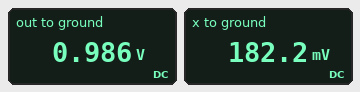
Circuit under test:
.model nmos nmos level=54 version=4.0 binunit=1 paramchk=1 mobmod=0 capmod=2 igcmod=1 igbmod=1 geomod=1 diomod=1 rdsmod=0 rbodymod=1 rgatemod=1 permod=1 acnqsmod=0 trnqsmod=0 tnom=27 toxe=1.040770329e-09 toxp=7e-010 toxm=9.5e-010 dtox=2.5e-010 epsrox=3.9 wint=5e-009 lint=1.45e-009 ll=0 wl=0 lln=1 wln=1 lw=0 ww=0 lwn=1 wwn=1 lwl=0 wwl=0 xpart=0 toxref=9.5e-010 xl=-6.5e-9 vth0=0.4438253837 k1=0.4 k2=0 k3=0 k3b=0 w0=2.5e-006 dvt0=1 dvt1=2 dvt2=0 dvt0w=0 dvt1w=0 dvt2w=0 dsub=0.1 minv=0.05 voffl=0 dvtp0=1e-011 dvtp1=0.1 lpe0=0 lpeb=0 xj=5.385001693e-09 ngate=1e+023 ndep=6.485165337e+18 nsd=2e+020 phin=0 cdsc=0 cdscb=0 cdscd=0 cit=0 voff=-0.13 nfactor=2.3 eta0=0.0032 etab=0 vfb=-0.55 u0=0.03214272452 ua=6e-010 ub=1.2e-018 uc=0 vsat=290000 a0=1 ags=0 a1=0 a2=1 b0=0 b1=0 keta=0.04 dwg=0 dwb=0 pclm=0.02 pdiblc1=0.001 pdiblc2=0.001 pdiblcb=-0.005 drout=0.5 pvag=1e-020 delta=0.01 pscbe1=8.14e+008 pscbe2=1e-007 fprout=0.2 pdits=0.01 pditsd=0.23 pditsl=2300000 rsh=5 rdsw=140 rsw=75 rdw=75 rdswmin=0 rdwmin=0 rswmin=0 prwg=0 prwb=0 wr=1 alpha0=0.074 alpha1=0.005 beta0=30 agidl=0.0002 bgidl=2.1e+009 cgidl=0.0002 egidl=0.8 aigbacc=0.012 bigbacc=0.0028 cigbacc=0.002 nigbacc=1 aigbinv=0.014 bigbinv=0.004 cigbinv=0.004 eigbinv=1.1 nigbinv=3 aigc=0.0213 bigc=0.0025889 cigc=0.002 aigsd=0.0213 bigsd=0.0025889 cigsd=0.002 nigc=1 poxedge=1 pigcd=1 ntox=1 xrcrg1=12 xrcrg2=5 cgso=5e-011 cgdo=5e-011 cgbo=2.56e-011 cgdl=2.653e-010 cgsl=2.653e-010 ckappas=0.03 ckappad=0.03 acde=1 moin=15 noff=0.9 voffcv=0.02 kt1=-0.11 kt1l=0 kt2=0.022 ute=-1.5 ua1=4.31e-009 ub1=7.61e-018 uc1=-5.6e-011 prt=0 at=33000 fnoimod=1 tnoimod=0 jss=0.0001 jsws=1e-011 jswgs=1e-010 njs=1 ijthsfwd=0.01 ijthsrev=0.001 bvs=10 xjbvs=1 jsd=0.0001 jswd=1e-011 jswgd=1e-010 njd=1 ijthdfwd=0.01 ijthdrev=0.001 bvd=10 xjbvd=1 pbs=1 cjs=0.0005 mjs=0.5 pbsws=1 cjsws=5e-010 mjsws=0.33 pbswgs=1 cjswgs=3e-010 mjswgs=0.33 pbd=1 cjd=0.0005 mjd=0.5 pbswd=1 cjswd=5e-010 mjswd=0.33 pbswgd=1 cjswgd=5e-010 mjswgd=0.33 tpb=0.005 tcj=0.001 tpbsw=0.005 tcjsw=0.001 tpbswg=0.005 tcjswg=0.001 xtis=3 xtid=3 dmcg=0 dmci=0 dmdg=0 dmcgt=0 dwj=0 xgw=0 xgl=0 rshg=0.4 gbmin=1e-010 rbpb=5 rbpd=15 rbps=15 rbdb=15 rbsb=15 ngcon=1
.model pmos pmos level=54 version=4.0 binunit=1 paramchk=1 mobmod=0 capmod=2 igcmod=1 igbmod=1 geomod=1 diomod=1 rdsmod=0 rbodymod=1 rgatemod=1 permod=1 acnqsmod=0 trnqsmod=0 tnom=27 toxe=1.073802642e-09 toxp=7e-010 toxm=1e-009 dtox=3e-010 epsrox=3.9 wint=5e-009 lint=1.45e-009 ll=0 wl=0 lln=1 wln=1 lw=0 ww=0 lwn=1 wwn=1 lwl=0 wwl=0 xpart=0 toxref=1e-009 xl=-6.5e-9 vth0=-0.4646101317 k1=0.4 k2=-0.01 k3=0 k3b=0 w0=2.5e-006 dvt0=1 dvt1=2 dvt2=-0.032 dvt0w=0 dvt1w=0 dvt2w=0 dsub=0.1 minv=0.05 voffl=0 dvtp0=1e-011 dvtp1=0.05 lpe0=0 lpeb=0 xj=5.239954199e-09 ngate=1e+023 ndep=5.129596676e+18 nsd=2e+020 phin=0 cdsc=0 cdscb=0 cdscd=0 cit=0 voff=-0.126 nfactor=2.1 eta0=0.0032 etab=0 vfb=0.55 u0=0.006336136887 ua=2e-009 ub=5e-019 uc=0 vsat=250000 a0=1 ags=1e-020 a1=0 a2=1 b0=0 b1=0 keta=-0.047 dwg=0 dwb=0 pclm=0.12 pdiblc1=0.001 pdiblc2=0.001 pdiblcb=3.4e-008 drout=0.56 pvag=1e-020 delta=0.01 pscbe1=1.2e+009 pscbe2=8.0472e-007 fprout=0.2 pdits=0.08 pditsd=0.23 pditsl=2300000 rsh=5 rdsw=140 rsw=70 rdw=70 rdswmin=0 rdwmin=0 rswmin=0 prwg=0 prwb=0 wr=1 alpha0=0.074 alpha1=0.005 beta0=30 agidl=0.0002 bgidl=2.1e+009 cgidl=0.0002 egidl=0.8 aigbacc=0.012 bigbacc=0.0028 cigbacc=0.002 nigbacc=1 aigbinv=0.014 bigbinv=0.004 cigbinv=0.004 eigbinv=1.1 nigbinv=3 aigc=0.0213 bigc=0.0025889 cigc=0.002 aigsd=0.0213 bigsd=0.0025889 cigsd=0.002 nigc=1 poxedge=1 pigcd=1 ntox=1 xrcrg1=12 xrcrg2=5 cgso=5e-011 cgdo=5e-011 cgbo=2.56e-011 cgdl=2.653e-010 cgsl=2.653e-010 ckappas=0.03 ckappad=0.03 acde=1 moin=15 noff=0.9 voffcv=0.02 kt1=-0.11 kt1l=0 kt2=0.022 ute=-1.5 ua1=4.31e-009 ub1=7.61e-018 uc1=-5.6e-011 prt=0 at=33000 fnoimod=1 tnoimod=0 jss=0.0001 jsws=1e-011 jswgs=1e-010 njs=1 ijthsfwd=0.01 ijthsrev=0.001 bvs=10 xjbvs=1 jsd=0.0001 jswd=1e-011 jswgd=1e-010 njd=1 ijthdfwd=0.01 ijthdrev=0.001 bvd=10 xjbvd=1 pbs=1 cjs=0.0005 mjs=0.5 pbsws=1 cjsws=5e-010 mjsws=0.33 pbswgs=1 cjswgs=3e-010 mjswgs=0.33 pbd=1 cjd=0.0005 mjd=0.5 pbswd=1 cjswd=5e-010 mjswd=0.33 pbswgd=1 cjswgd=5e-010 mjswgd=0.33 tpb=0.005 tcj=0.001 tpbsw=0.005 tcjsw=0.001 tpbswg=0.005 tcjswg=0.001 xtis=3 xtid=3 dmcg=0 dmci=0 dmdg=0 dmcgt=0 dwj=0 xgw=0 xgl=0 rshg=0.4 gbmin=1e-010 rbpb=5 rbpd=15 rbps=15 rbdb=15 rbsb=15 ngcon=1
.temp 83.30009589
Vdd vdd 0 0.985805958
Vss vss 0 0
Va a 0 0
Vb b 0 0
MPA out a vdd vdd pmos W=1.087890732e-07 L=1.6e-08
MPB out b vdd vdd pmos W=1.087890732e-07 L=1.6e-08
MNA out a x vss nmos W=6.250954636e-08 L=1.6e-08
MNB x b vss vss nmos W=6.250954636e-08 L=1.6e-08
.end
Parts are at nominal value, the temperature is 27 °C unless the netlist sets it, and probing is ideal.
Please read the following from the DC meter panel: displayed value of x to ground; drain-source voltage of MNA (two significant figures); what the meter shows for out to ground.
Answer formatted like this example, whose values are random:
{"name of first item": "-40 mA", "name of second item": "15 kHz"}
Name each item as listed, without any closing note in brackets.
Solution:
{"displayed value of x to ground": "182.2 mV", "drain-source voltage of MNA": "800 mV", "what the meter shows for out to ground": "0.986 V"}
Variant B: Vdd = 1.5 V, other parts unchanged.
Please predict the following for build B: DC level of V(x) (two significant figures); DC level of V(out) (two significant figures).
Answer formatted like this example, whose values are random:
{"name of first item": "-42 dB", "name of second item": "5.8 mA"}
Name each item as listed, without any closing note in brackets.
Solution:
{"DC level of V(x)": "290 mV", "DC level of V(out)": "1.5 V"}
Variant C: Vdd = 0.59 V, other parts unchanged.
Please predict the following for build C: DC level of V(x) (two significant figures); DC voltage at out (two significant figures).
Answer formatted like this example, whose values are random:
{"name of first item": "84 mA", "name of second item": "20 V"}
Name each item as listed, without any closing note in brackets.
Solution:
{"DC level of V(x)": "110 mV", "DC voltage at out": "590 mV"}
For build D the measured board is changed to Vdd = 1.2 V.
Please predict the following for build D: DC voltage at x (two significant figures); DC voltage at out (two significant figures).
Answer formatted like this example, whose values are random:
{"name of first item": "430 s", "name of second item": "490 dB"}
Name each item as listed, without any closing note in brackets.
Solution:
{"DC voltage at x": "230 mV", "DC voltage at out": "1.2 V"}
